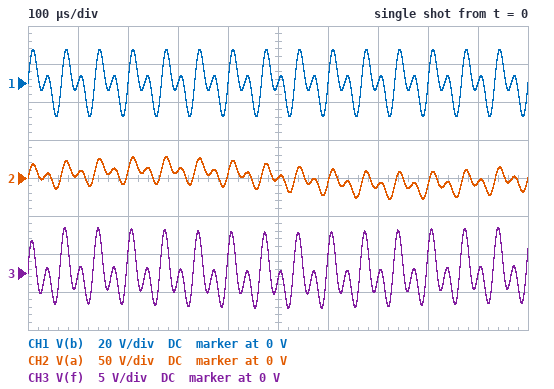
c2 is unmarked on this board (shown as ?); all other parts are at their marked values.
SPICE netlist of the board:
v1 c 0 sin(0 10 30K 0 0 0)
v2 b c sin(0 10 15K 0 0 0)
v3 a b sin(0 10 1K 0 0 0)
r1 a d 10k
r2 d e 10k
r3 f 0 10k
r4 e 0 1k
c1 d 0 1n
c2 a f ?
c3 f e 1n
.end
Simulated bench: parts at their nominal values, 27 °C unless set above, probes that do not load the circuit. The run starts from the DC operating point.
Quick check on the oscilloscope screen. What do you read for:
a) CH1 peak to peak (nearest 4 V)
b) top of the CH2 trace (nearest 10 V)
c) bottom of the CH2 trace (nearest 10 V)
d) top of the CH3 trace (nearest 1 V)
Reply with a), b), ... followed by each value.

a) 36 V
b) 30 V
c) -30 V
d) 6 V
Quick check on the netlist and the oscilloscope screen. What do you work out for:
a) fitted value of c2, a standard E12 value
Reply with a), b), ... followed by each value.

a) 470 pF
